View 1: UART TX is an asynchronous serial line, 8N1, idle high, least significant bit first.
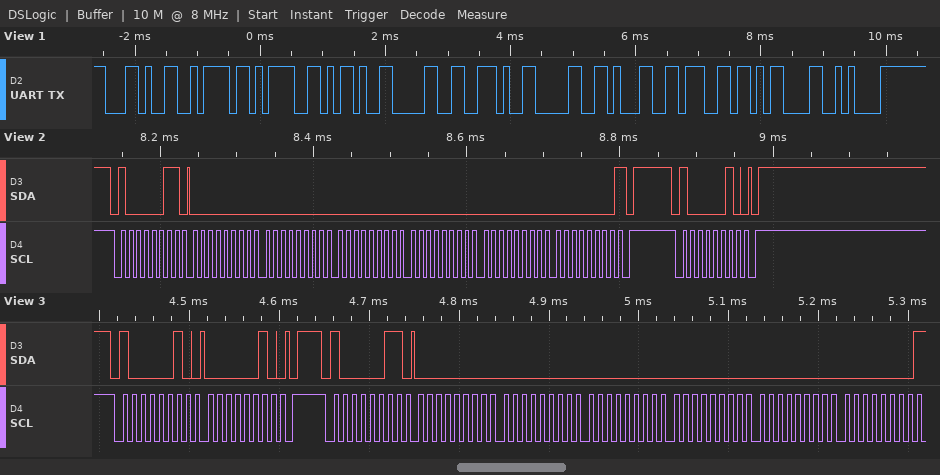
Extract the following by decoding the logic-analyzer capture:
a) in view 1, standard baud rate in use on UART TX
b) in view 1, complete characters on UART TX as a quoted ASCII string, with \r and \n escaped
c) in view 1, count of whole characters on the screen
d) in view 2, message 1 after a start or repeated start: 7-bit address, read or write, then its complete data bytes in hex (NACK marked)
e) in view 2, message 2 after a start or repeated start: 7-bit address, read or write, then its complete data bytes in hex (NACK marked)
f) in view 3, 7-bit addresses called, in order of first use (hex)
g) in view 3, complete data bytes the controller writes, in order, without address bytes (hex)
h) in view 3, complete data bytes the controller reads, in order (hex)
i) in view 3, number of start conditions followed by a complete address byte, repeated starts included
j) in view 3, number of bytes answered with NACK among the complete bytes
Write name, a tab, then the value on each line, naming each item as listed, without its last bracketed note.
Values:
in view 1, standard baud rate in use on UART TX	9600 baud
in view 1, complete characters on UART TX as a quoted ASCII string, with \r and \n escaped	",z=-0.01g\r\n"
in view 1, count of whole characters on the screen	11
in view 2, message 1 after a start or repeated start: 7-bit address, read or write, then its complete data bytes in hex	0x41 read: 00 00 00 00 00 00 NACK
in view 2, message 2 after a start or repeated start: 7-bit address, read or write, then its complete data bytes in hex	0x41 write
in view 3, 7-bit addresses called, in order of first use	0x41
in view 3, complete data bytes the controller writes, in order, without address bytes	02
in view 3, complete data bytes the controller reads, in order	00 00 00 00 00 00
in view 3, number of start conditions followed by a complete address byte, repeated starts included	2
in view 3, number of bytes answered with NACK among the complete bytes	1
